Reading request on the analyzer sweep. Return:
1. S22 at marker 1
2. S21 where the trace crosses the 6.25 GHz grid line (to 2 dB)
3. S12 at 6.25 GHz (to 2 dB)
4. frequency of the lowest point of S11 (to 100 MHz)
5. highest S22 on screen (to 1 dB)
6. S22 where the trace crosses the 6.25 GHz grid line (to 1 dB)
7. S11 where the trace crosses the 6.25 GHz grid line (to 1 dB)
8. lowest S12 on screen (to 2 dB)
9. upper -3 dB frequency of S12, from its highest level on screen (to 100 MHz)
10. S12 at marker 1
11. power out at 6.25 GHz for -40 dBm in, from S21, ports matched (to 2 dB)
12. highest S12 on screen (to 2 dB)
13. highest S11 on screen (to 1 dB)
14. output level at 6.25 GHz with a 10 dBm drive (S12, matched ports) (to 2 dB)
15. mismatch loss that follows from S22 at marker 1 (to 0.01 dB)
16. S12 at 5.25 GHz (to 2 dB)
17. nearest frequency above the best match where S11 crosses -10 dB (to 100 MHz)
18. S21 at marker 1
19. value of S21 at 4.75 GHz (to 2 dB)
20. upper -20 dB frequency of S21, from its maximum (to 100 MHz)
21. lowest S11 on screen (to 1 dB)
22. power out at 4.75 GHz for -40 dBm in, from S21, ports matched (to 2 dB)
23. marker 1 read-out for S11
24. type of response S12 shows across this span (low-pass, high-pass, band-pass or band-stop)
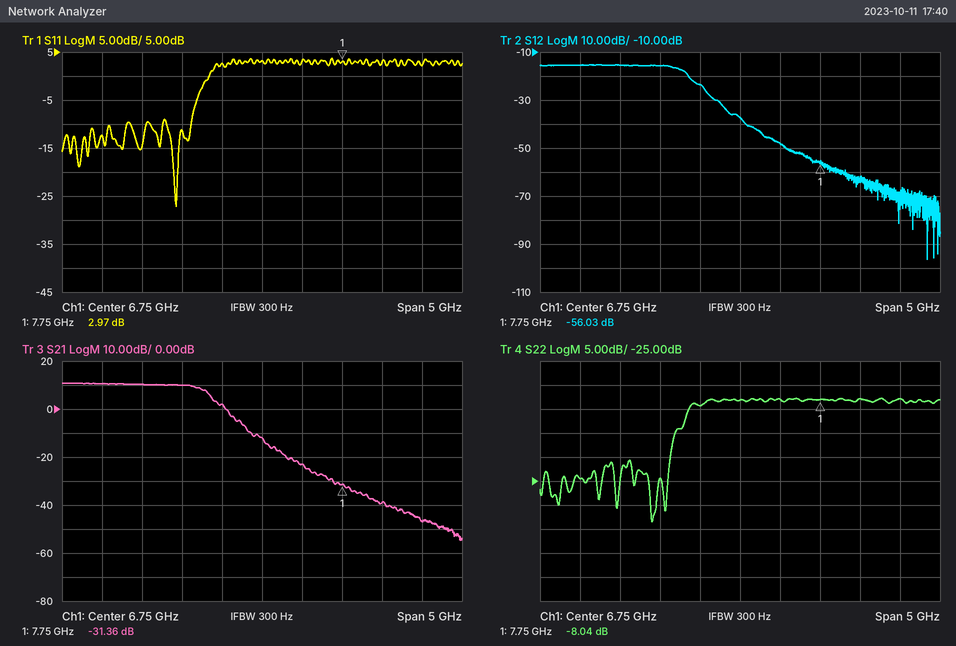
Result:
-8.04 dB
2 dB
-24 dB
5.7 GHz
-8 dB
-9 dB
3 dB
-96 dB
6.1 GHz
-56.03 dB
-38 dBm
-16 dB
4 dB
-14 dBm
0.74 dB
-16 dB
5.9 GHz
-31.36 dB
10 dB
6.6 GHz
-27 dB
-30 dBm
2.97 dB
low-pass
